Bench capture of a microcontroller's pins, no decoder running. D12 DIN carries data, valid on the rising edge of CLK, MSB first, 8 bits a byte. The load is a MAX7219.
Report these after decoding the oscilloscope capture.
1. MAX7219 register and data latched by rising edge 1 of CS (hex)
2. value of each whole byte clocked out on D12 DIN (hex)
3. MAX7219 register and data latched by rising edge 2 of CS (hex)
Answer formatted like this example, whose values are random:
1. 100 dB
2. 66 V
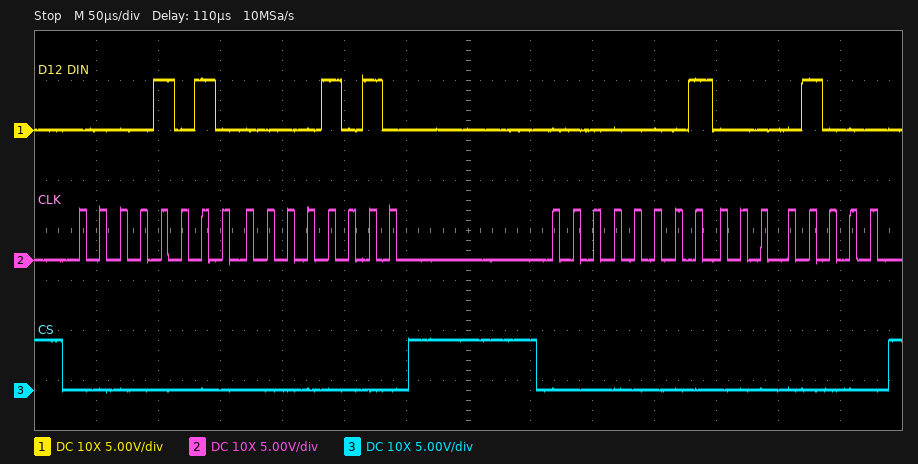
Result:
1. register 0xA, data 0x0A
2. 0x0A 0x0A 0x01 0x08
3. register 0x1, data 0x08
